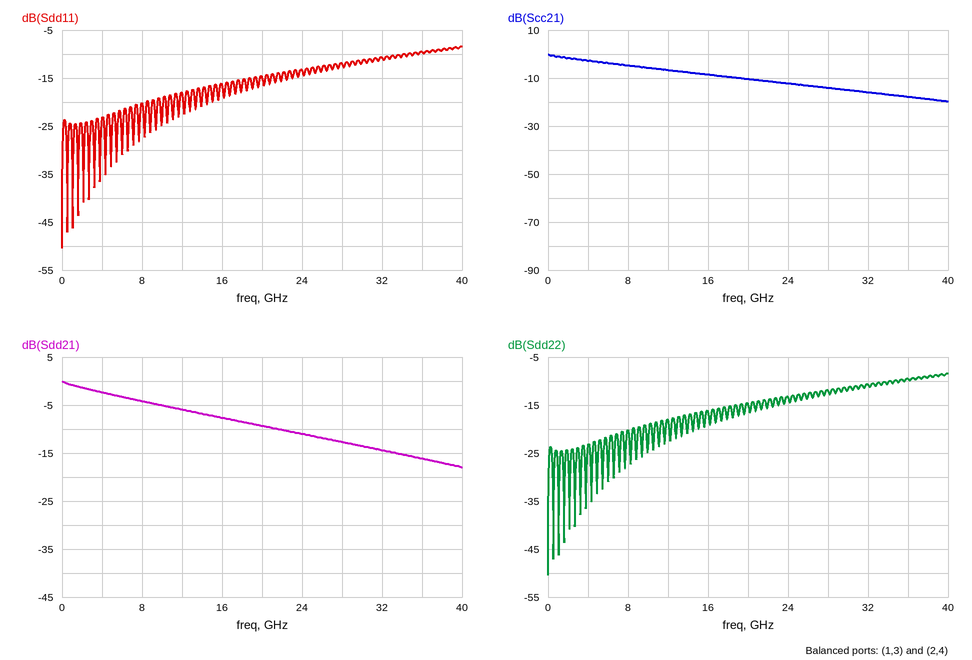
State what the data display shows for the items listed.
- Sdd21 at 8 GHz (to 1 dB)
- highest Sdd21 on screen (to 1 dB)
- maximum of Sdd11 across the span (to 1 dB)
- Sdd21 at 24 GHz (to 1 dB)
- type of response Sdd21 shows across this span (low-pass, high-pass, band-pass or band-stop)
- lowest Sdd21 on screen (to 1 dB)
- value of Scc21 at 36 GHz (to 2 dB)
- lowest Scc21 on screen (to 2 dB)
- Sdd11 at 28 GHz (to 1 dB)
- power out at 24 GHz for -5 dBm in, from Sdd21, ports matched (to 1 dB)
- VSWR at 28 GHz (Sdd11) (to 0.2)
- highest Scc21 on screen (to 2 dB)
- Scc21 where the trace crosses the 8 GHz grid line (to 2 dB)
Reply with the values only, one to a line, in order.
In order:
-4 dB
0 dB
-8 dB
-11 dB
low-pass
-18 dB
-18 dB
-20 dB
-12 dB
-16 dBm
1.6
0 dB
-4 dB
